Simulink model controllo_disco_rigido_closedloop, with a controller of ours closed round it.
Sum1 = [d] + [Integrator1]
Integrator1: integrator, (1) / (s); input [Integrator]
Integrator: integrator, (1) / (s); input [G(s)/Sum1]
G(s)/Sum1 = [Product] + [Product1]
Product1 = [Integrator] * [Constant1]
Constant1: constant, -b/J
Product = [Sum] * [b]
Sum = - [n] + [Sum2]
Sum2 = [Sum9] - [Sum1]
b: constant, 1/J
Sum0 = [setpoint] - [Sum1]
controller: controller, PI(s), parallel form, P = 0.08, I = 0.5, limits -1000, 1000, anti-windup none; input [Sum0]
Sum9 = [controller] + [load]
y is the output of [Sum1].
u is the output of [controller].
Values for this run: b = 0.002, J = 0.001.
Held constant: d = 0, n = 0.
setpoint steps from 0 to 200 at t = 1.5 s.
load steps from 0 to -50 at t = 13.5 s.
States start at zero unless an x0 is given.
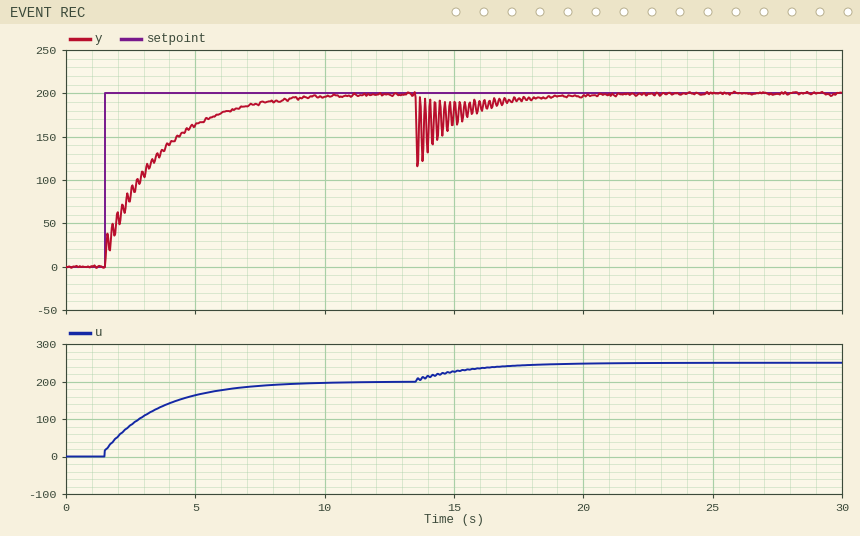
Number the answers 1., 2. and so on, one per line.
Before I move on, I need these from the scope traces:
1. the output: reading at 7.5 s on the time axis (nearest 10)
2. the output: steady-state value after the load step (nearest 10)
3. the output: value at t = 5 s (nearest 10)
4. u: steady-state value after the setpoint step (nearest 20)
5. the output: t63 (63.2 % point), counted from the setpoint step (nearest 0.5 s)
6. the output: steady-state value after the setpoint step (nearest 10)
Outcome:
1. 190
2. 200
3. 160
4. 200
5. 2.0 s
6. 200
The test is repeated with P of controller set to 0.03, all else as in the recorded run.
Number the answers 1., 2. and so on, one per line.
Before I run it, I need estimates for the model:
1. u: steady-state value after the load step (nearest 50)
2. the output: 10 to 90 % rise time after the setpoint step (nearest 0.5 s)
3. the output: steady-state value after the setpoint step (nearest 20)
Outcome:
1. 250
2. 4.5 s
3. 200
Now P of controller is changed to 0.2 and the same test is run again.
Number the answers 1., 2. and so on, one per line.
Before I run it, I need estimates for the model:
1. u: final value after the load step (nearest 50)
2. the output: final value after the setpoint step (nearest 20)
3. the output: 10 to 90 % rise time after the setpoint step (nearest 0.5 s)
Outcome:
1. 250
2. 200
3. 5.0 s
